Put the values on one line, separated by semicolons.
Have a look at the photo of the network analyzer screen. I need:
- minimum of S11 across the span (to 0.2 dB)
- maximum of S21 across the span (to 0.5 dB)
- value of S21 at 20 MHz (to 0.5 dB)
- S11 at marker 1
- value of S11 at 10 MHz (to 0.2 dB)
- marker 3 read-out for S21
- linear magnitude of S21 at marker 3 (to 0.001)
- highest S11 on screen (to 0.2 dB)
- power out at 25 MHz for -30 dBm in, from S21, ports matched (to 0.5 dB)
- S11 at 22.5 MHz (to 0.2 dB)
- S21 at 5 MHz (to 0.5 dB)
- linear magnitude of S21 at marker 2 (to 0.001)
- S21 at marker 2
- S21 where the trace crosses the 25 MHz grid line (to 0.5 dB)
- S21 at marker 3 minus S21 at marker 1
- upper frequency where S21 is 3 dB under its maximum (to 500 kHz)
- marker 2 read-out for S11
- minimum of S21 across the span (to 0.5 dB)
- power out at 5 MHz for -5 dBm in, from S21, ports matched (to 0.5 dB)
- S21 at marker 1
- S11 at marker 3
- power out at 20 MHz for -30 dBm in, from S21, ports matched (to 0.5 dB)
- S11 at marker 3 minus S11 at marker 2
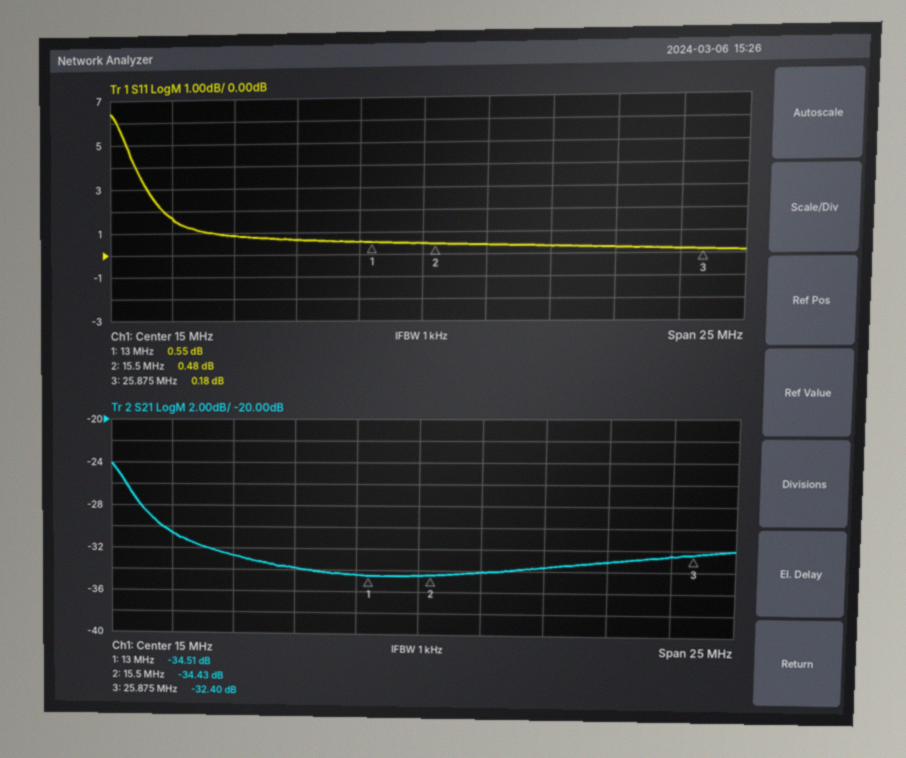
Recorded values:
0.2 dB; -24.0 dB; -33.5 dB; 0.55 dB; 0.6 dB; -32.40 dB; 0.024; 6.4 dB; -62.5 dBm; 0.2 dB; -30.5 dB; 0.019; -34.43 dB; -32.5 dB; 2.11 dB; 3.5 MHz; 0.48 dB; -34.5 dB; -35.5 dBm; -34.51 dB; 0.18 dB; -63.5 dBm; -0.30 dB
